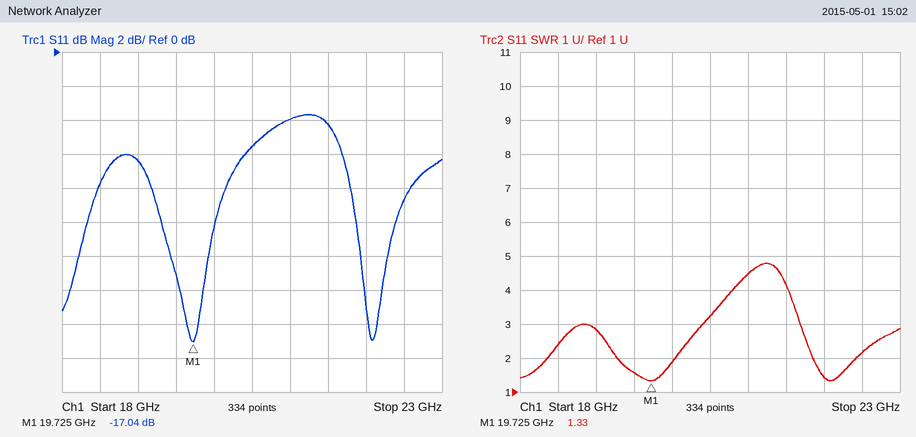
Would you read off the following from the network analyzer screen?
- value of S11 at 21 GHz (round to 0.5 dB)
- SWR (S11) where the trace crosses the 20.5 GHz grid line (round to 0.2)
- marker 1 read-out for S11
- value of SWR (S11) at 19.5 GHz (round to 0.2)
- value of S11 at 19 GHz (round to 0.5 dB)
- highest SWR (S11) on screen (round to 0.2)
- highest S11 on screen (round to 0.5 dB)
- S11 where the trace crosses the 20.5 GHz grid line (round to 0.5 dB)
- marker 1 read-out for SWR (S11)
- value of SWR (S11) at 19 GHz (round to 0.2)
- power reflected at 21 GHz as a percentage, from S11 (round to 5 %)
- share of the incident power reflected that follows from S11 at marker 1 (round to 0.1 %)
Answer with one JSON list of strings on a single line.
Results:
["-4.0 dB", "3.2", "-17.04 dB", "1.6", "-6.5 dB", "4.8", "-3.5 dB", "-5.5 dB", "1.33", "2.8", "40 %", "2.0 %"]
